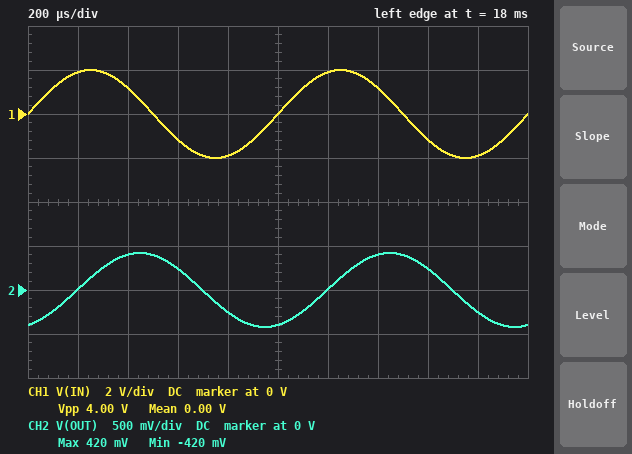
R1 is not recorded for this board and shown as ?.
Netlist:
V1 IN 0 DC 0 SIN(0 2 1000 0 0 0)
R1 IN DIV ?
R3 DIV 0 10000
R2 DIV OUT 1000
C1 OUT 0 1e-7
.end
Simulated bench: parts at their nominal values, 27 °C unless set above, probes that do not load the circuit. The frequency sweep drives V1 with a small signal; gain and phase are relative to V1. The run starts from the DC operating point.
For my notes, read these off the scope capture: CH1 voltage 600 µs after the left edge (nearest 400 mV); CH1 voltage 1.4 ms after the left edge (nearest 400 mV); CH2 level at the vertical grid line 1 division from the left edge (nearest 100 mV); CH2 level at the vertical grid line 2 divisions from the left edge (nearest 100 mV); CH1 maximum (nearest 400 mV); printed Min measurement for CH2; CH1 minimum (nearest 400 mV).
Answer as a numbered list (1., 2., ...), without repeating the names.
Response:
1. -1.2 V
2. 1.2 V
3. 0 V
4. 400 mV
5. 2.0 V
6. -420 mV
7. -2.0 V
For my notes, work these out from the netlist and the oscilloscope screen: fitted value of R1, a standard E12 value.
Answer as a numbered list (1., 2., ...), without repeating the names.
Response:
1. 5.6 kΩ
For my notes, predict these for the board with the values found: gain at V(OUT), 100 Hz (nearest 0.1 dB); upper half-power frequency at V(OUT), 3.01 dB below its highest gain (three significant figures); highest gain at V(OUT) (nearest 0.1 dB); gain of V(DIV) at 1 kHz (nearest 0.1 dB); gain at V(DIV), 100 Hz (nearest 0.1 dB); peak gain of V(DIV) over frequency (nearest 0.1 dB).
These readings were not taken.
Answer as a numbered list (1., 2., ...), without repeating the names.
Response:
1. -4.2 dB
2. 347 Hz
3. -3.9 dB
4. -12.1 dB
5. -4.2 dB
6. -3.9 dB
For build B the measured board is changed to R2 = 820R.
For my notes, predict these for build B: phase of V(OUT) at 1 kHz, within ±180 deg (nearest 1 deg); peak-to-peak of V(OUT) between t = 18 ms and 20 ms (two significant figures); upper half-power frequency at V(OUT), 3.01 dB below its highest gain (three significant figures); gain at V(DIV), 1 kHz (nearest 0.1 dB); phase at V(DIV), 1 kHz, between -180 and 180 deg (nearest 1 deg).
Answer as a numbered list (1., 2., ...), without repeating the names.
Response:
1. -70 deg
2. 870 mV
3. 361 Hz
4. -12.2 dB
5. -43 deg
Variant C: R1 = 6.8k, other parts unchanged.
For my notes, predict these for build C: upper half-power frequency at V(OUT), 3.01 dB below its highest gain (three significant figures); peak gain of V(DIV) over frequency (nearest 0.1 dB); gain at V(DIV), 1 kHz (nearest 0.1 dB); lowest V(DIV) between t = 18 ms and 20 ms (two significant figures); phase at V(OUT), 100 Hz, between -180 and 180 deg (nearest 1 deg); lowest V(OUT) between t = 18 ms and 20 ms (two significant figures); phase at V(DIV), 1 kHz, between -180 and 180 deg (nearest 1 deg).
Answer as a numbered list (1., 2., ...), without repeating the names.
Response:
1. 315 Hz
2. -4.5 dB
3. -13.5 dB
4. -420 mV
5. -18 deg
6. -360 mV
7. -40 deg
